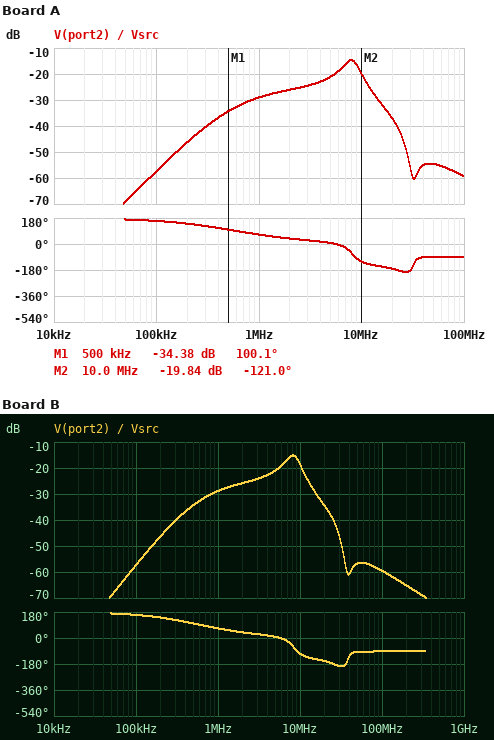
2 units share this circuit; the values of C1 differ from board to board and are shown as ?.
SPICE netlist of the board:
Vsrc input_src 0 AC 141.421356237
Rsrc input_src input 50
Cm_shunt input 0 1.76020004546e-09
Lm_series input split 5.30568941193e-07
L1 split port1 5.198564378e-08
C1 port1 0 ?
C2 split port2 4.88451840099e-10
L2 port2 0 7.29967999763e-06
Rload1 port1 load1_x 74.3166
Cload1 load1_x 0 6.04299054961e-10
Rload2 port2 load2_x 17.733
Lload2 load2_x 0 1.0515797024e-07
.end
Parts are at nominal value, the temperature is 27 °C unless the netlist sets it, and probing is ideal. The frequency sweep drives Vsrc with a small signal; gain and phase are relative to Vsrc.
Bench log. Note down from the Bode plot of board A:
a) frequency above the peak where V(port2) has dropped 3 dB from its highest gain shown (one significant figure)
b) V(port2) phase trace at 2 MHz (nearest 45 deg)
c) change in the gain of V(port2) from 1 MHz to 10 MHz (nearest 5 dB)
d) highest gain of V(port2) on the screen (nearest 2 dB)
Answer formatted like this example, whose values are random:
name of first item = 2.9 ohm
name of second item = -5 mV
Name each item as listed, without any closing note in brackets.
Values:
frequency above the peak where V(port2) has dropped 3 dB from its highest gain shown = 9 MHz
V(port2) phase trace at 2 MHz = 45 deg
change in the gain of V(port2) from 1 MHz to 10 MHz = 10 dB
highest gain of V(port2) on the screen = -14 dB
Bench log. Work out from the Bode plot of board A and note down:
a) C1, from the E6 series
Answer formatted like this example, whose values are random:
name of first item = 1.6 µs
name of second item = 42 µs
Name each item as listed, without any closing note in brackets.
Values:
C1, from the E6 series = 470 pF
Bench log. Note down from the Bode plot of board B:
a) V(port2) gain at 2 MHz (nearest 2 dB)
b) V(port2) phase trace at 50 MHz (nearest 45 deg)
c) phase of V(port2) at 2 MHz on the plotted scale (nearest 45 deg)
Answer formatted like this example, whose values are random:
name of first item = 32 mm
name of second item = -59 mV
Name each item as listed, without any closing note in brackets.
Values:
V(port2) gain at 2 MHz = -26 dB
V(port2) phase trace at 50 MHz = -90 deg
phase of V(port2) at 2 MHz on the plotted scale = 45 deg
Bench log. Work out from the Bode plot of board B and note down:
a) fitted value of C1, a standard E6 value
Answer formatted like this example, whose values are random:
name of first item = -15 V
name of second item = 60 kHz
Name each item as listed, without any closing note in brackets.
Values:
fitted value of C1, a standard E6 value = 330 pF
